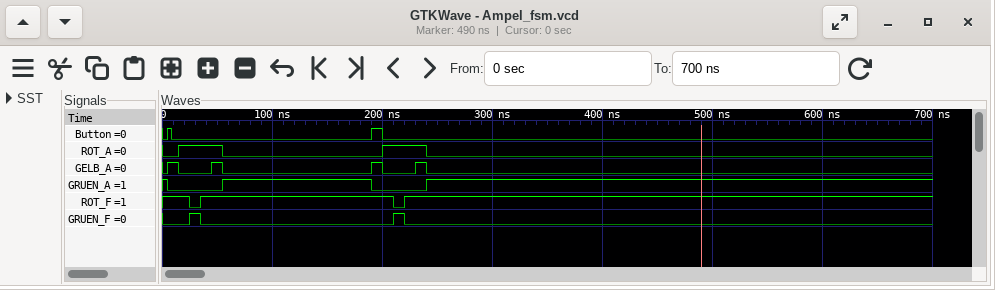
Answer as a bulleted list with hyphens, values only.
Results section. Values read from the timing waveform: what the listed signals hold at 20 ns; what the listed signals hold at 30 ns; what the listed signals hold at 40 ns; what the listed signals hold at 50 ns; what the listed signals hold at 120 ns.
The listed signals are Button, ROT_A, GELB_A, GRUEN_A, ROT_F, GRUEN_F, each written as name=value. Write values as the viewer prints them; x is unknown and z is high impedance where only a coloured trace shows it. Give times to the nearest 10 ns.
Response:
- Button=0, ROT_A=1, GELB_A=0, GRUEN_A=0, ROT_F=1, GRUEN_F=0
- Button=0, ROT_A=1, GELB_A=0, GRUEN_A=0, ROT_F=0, GRUEN_F=1
- Button=0, ROT_A=1, GELB_A=0, GRUEN_A=0, ROT_F=1, GRUEN_F=0
- Button=0, ROT_A=1, GELB_A=1, GRUEN_A=0, ROT_F=1, GRUEN_F=0
- Button=0, ROT_A=0, GELB_A=0, GRUEN_A=1, ROT_F=1, GRUEN_F=0
